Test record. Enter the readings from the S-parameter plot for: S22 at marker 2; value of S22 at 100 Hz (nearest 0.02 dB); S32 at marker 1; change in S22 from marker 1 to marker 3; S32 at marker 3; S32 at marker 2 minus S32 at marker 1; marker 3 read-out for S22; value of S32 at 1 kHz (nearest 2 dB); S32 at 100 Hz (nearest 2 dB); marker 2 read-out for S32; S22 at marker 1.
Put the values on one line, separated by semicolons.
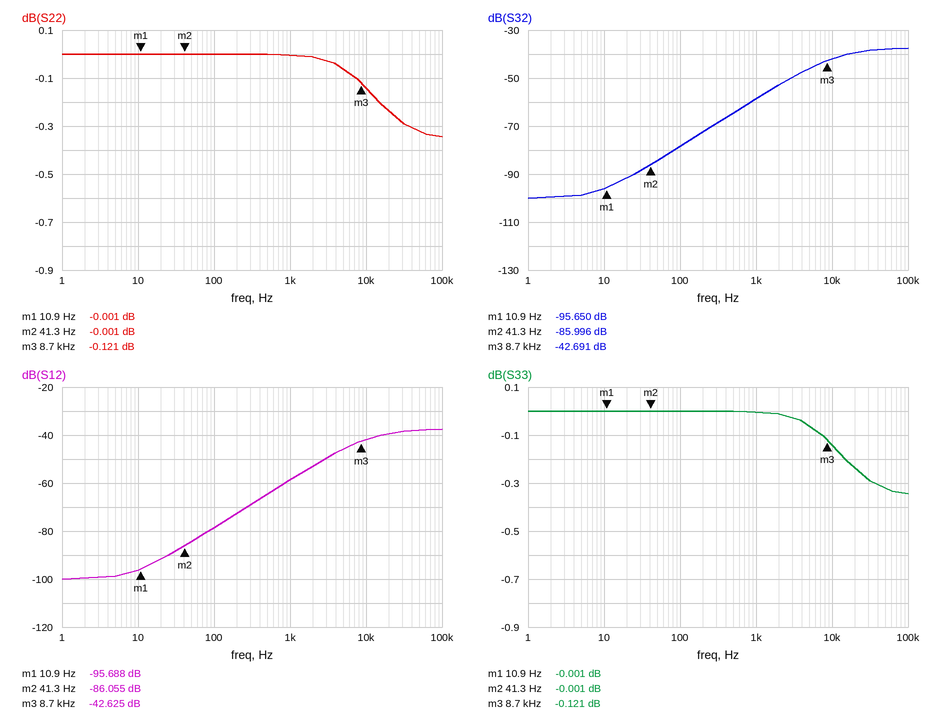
-0.001 dB; 0.00 dB; -95.650 dB; -0.120 dB; -42.691 dB; 9.654 dB; -0.121 dB; -58 dB; -78 dB; -85.996 dB; -0.001 dB
